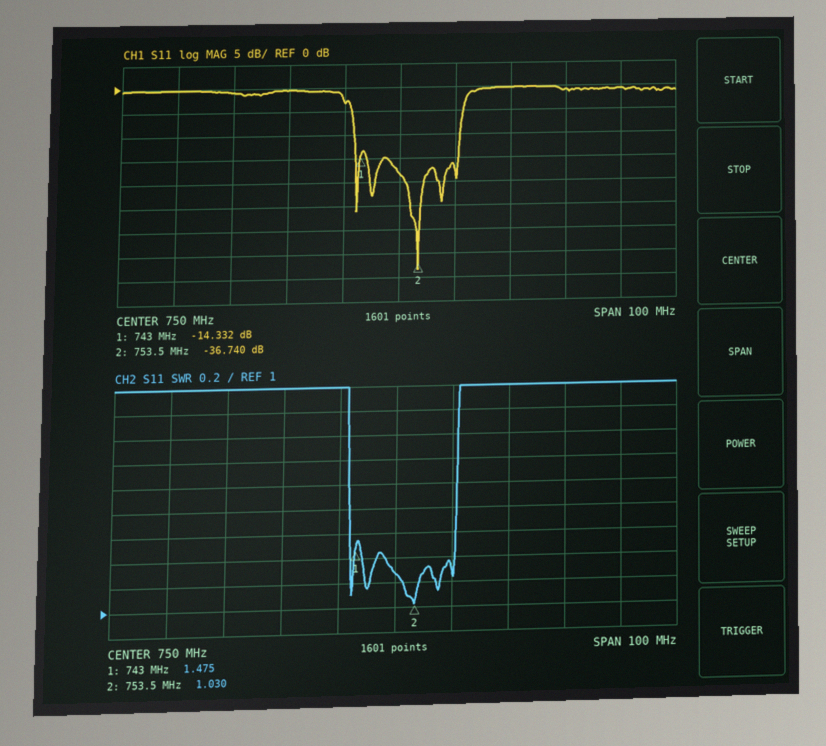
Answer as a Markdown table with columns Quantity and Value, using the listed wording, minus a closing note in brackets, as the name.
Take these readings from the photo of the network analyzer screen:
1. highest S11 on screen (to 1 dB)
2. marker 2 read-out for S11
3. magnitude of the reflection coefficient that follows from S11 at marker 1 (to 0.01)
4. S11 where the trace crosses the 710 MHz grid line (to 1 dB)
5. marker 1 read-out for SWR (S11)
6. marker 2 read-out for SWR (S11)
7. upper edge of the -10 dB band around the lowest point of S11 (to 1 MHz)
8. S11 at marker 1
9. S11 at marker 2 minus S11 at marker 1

| Quantity | Value |
|---|---|
| highest S11 on screen | 0 dB |
| marker 2 read-out for S11 | -36.740 dB |
| magnitude of the reflection coefficient that follows from S11 at marker 1 | 0.19 |
| S11 where the trace crosses the 710 MHz grid line | 0 dB |
| marker 1 read-out for SWR | 1.475 |
| marker 2 read-out for SWR | 1.030 |
| upper edge of the -10 dB band around the lowest point of S11 | 761 MHz |
| S11 at marker 1 | -14.332 dB |
| S11 at marker 2 minus S11 at marker 1 | -22.408 dB |
